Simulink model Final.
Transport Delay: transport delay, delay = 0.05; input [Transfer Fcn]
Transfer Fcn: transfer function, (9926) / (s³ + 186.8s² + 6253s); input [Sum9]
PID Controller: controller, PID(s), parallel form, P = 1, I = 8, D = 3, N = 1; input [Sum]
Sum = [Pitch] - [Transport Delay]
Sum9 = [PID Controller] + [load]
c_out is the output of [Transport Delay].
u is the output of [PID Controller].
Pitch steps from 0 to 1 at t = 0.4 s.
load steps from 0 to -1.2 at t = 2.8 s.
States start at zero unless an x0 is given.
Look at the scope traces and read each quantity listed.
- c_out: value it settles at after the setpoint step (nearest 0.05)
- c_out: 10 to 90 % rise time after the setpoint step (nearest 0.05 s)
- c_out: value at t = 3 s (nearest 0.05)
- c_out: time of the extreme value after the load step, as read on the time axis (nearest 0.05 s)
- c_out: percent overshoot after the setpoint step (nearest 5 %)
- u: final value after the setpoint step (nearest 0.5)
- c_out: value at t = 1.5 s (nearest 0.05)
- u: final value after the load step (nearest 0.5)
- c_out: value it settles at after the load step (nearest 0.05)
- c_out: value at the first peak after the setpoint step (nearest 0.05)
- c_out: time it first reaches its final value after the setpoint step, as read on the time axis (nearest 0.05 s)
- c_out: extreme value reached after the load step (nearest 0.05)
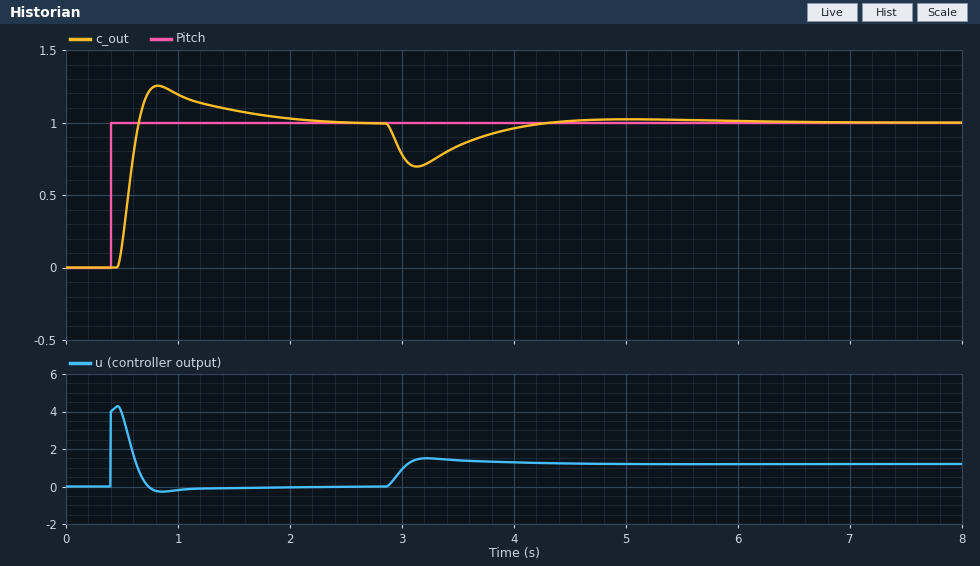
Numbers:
1.00
0.15 s
0.80
3.15 s
25 %
0.0
1.10
1.0
1.00
1.25
0.65 s
0.70
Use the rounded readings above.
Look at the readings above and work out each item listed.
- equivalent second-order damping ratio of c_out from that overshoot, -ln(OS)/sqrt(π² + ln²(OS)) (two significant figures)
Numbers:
0.40
